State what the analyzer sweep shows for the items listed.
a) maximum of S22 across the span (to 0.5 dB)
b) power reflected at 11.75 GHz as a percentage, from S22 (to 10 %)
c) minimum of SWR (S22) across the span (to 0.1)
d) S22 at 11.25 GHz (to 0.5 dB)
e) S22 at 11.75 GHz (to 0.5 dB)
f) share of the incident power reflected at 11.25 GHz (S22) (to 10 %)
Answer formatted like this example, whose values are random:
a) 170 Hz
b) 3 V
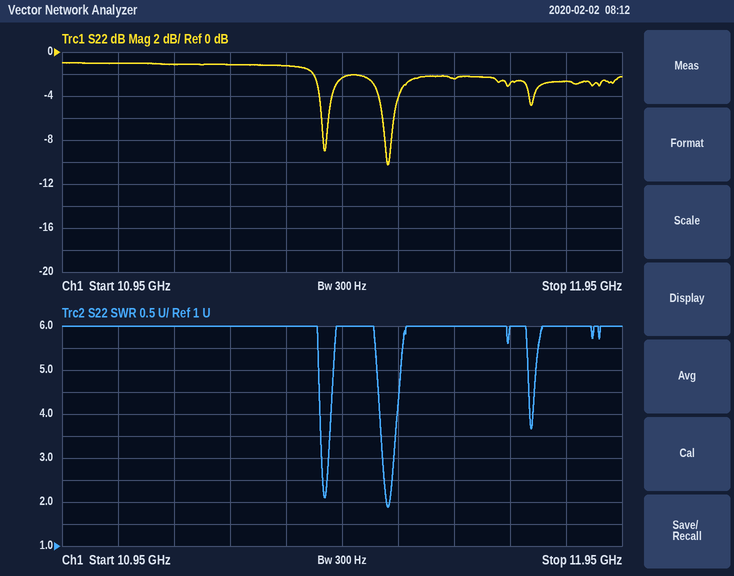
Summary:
a) -1.0 dB
b) 50 %
c) 1.9
d) -1.0 dB
e) -3.0 dB
f) 80 %
